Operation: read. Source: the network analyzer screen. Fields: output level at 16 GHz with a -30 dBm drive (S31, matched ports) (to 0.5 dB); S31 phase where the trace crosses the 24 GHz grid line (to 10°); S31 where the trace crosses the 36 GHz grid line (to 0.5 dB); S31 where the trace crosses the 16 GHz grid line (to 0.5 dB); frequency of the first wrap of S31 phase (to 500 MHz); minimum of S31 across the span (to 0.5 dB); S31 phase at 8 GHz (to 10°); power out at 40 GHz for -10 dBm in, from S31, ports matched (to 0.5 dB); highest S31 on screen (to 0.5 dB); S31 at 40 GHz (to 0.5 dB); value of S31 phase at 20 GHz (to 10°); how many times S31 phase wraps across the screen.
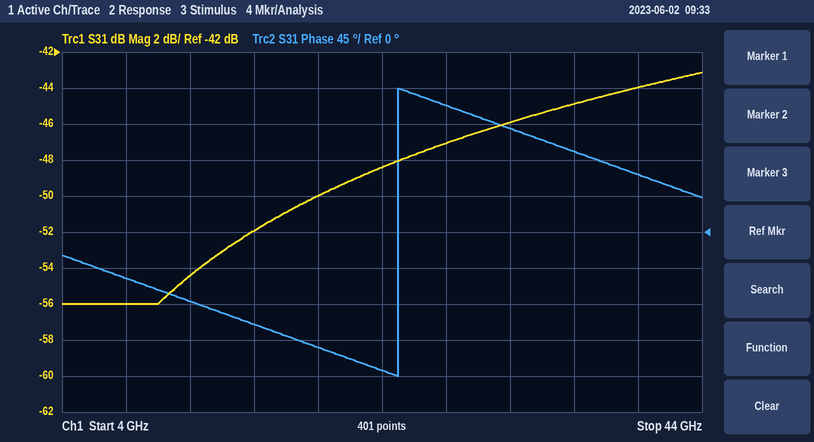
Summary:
-82.0 dBm
-170°
-45.0 dB
-52.0 dB
25.0 GHz
-56.0 dB
-60°
-54.0 dBm
-43.0 dB
-44.0 dB
-140°
1
